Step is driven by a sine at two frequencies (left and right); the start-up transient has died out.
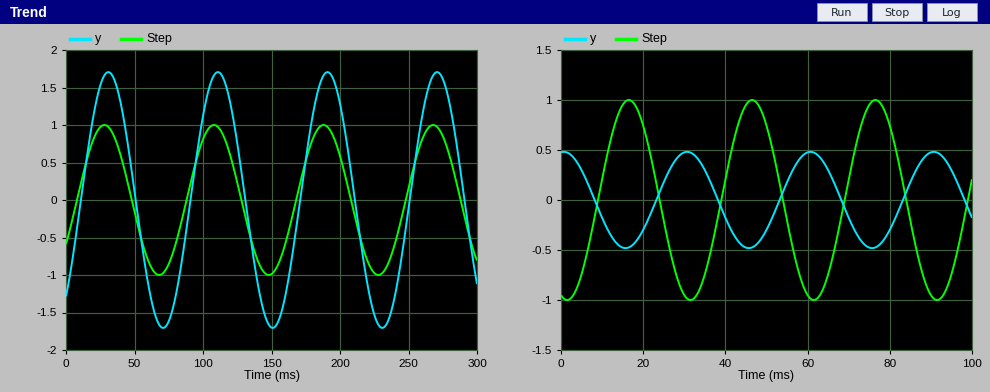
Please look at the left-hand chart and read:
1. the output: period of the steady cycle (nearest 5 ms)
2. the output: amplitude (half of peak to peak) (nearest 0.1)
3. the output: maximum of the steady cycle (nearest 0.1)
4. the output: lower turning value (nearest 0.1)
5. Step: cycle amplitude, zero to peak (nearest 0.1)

80 ms
1.7
1.7
-1.7
1.0
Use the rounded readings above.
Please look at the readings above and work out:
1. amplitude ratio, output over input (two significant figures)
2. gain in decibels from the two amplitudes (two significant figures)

1.7
4.6 dB
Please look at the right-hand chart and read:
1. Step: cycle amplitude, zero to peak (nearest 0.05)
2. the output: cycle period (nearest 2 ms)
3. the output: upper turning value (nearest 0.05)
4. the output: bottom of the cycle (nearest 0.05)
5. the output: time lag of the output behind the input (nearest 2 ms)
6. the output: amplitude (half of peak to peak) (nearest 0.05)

1.00
30 ms
0.50
-0.50
14 ms
0.50
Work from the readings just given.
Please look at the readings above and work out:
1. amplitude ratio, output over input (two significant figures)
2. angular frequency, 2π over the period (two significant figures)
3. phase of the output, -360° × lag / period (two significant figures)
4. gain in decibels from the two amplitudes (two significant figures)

0.50
0.21 rad/ms
-170°
-6.0 dB
